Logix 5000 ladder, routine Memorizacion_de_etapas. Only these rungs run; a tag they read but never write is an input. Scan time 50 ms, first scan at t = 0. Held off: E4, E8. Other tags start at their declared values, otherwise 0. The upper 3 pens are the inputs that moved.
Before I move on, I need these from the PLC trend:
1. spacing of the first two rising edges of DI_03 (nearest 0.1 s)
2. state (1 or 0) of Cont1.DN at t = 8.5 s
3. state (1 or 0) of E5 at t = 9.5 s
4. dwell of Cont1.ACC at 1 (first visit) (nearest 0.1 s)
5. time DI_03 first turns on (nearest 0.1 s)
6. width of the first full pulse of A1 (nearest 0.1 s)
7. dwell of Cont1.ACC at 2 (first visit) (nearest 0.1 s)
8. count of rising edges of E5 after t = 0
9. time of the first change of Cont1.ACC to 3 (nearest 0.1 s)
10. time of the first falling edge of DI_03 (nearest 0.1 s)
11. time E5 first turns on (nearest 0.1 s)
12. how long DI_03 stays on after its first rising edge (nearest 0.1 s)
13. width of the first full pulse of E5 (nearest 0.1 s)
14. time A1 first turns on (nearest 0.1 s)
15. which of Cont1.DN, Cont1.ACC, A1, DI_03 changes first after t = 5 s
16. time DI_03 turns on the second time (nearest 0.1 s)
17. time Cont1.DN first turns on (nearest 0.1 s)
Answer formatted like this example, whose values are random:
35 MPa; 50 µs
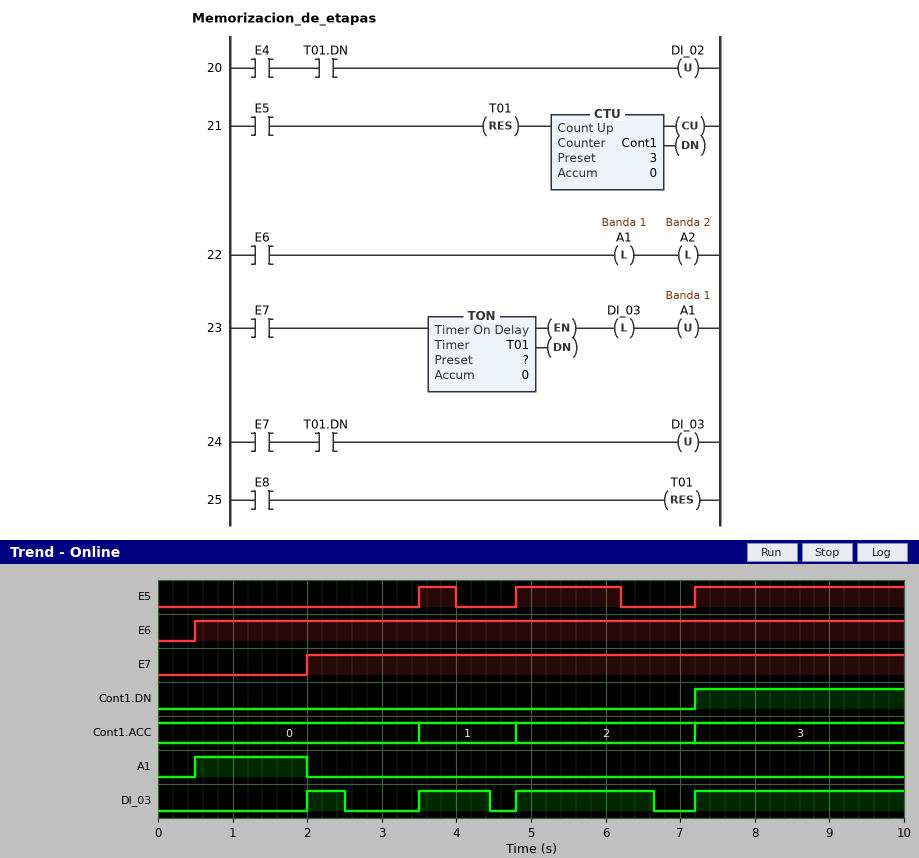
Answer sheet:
1.5 s; 1; 1; 1.3 s; 2.0 s; 1.5 s; 2.4 s; 3; 7.2 s; 2.5 s; 3.5 s; 0.5 s; 0.5 s; 0.5 s; DI_03; 3.5 s; 7.2 s
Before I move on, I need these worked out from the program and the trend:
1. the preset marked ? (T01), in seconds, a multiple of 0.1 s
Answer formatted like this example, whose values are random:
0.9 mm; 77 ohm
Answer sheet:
0.5 s
